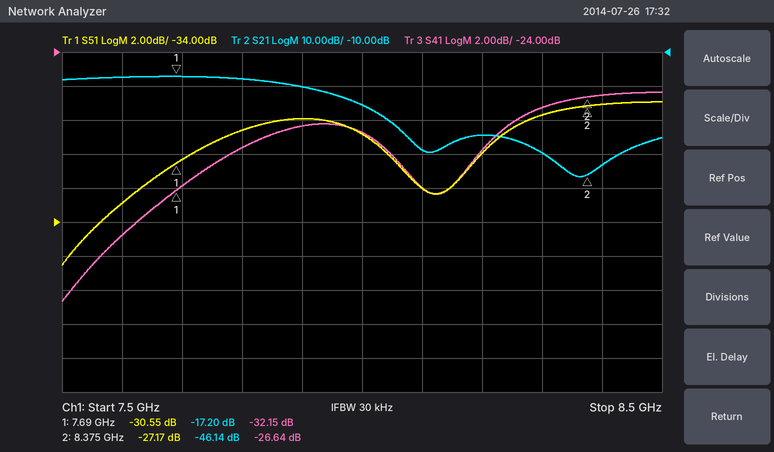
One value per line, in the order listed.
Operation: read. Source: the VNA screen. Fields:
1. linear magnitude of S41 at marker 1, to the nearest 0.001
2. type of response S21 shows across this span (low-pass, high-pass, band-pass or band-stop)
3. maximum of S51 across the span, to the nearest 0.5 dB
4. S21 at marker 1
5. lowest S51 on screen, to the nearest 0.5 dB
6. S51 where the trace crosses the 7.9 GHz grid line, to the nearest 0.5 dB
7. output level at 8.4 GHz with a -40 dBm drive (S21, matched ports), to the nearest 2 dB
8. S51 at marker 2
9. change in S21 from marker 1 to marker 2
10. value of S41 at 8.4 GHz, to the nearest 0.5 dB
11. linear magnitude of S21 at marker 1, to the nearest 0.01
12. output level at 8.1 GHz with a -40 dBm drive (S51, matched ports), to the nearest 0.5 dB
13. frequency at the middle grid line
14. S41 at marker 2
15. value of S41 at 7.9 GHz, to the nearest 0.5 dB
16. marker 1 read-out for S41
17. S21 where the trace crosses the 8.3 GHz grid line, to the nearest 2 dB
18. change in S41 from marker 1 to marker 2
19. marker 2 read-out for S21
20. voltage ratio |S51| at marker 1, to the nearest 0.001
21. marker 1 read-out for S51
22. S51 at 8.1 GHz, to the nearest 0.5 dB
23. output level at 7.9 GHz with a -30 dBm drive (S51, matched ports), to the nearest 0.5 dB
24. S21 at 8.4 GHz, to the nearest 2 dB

0.025
low-pass
-27.0 dB
-17.20 dB
-36.5 dB
-28.0 dB
-84 dBm
-27.17 dB
-28.94 dB
-26.5 dB
0.14
-72.0 dBm
8 GHz
-26.64 dB
-28.5 dB
-32.15 dB
-40 dB
5.51 dB
-46.14 dB
0.030
-30.55 dB
-32.0 dB
-58.0 dBm
-44 dB
